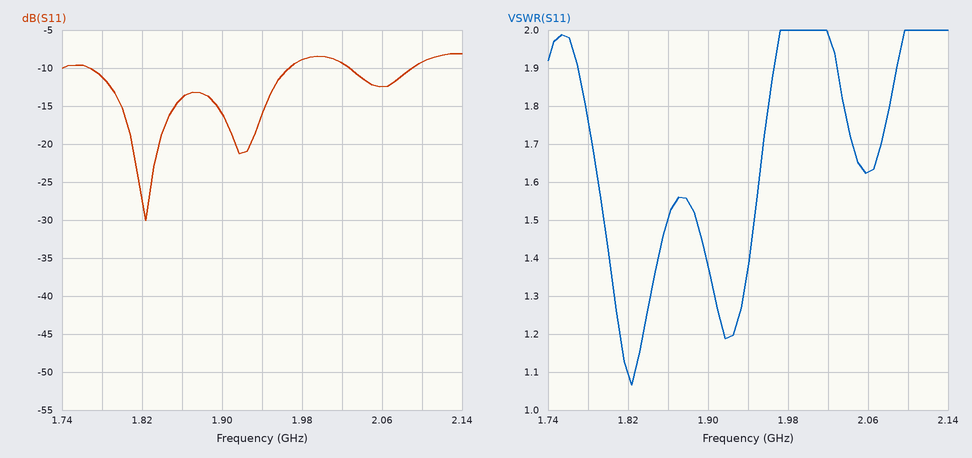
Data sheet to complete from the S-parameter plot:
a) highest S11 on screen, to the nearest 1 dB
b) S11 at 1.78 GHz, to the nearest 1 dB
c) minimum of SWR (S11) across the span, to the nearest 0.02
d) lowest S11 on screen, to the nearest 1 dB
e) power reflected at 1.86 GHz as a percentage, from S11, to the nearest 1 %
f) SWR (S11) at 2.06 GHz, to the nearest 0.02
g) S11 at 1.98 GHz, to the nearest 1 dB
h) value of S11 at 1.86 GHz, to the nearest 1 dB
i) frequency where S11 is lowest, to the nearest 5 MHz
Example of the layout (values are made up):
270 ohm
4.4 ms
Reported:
-8 dB
-11 dB
1.06
-30 dB
4 %
1.62
-9 dB
-14 dB
1.825 GHz
